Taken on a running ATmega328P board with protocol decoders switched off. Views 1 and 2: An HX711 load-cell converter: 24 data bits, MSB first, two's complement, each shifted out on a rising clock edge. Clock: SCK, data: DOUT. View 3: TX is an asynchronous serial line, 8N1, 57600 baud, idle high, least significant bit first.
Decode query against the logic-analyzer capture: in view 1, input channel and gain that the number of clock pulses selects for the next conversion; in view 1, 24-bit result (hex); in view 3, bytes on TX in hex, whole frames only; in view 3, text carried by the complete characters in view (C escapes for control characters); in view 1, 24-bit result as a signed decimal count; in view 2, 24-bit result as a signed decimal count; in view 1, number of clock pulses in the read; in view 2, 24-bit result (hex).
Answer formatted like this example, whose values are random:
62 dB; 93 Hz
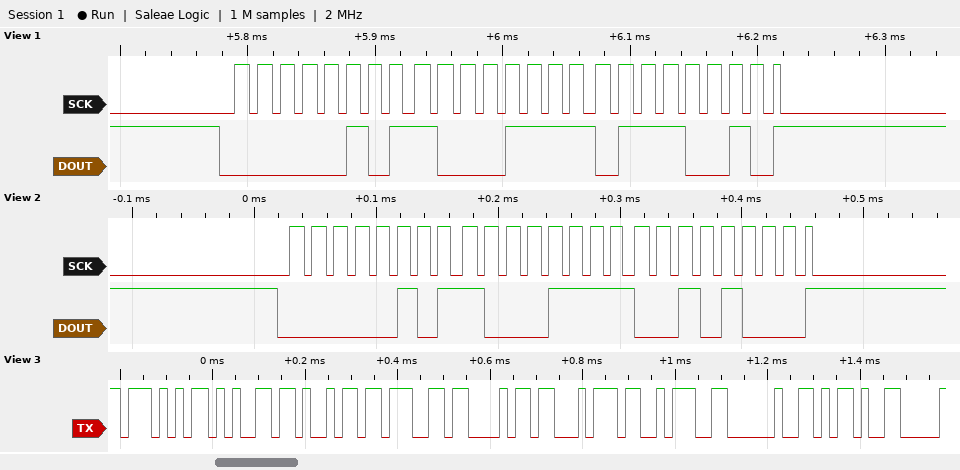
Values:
channel A, gain 128; 0x058F72; 57 65 69 67 68 74 3A 20 2D; "Weight: -"; 364402; 364328; 25; 0x058F28
